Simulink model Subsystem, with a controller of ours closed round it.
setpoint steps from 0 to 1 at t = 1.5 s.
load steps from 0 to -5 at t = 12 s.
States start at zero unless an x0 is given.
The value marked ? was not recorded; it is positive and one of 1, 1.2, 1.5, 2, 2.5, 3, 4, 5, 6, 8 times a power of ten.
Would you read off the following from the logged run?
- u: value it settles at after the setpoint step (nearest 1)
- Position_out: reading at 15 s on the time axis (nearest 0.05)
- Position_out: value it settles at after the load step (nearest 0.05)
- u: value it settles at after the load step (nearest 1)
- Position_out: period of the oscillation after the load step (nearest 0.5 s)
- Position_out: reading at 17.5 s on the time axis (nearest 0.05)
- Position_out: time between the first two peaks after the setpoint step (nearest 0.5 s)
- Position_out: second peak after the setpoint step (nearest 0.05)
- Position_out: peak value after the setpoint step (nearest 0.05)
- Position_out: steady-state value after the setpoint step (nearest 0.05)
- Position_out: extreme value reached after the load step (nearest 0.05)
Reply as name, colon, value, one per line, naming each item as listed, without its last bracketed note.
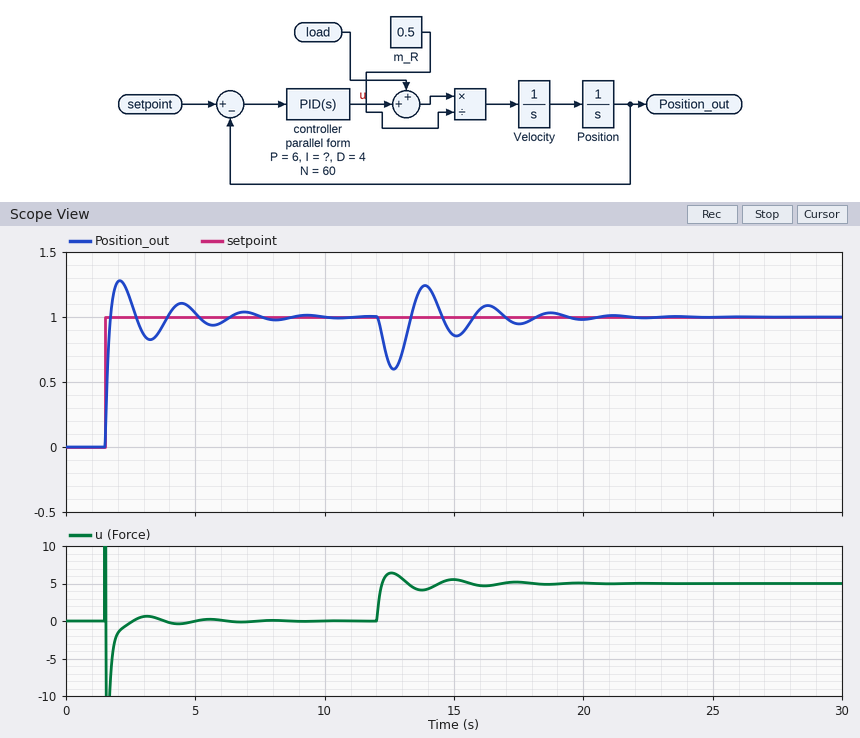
u: value it settles at after the setpoint step: 0
Position_out: reading at 15 s on the time axis: 0.85
Position_out: value it settles at after the load step: 1.00
u: value it settles at after the load step: 5
Position_out: period of the oscillation after the load step: 2.5 s
Position_out: reading at 17.5 s on the time axis: 0.95
Position_out: time between the first two peaks after the setpoint step: 2.5 s
Position_out: second peak after the setpoint step: 1.10
Position_out: peak value after the setpoint step: 1.30
Position_out: steady-state value after the setpoint step: 1.00
Position_out: extreme value reached after the load step: 0.60
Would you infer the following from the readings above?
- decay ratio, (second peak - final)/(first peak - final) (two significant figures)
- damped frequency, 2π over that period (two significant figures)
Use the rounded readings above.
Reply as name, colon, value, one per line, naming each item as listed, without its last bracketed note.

decay ratio, (second peak - final)/(first peak - final): 0.33
damped frequency, 2π over that period: 2.5 rad/s
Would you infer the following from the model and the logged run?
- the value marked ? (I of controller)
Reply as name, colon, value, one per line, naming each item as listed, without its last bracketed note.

the value marked ?: 25
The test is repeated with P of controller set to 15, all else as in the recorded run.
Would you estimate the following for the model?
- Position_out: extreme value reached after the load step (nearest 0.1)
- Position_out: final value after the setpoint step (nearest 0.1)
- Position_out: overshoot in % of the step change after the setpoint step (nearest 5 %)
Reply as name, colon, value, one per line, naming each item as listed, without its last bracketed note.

Position_out: extreme value reached after the load step: 0.7
Position_out: final value after the setpoint step: 1.0
Position_out: overshoot in % of the step change after the setpoint step: 30 %
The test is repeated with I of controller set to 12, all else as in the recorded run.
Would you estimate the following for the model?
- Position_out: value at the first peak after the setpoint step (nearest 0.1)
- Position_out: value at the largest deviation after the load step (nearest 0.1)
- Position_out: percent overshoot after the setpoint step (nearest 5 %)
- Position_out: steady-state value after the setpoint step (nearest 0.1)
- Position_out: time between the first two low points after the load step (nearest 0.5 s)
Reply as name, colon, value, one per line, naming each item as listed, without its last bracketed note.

Position_out: value at the first peak after the setpoint step: 1.2
Position_out: value at the largest deviation after the load step: 0.5
Position_out: percent overshoot after the setpoint step: 20 %
Position_out: steady-state value after the setpoint step: 1.0
Position_out: time between the first two low points after the load step: 3.5 s
